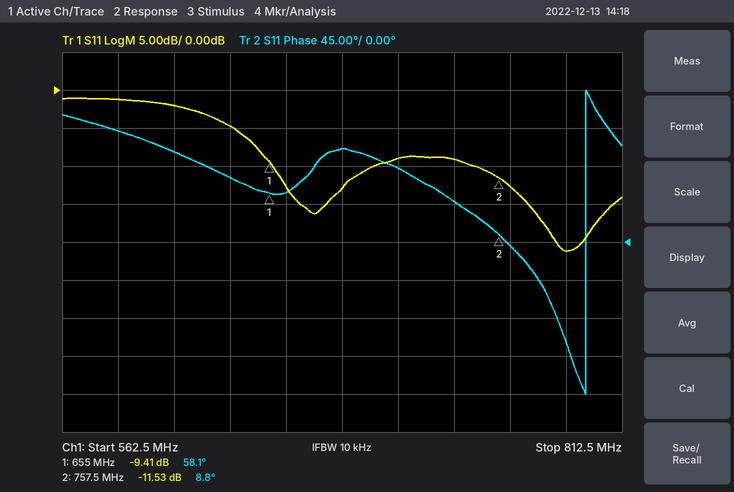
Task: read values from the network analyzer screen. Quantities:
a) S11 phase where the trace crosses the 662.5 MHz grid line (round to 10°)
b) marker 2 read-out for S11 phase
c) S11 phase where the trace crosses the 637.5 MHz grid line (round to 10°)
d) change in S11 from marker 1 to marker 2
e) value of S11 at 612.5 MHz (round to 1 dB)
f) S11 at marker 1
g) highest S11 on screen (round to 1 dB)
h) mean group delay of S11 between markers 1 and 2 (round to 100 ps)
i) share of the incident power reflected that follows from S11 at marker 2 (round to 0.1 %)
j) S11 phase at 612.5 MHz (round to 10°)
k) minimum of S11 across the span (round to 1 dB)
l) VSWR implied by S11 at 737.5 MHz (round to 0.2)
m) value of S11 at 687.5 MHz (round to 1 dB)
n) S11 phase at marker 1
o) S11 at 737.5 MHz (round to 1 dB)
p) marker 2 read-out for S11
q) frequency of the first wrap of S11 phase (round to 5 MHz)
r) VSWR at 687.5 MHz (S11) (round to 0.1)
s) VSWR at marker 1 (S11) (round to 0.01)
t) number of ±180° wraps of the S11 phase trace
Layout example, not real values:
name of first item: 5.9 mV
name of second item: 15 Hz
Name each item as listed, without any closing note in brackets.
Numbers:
S11 phase where the trace crosses the 662.5 MHz grid line: 60°
marker 2 read-out for S11 phase: 8.8°
S11 phase where the trace crosses the 637.5 MHz grid line: 80°
change in S11 from marker 1 to marker 2: -2.12 dB
value of S11 at 612.5 MHz: -2 dB
S11 at marker 1: -9.41 dB
highest S11 on screen: -1 dB
mean group delay of S11 between markers 1 and 2: 1.3 ns
share of the incident power reflected that follows from S11 at marker 2: 7.0 %
S11 phase at 612.5 MHz: 110°
minimum of S11 across the span: -21 dB
VSWR implied by S11 at 737.5 MHz: 2.0
value of S11 at 687.5 MHz: -13 dB
S11 phase at marker 1: 58.1°
S11 at 737.5 MHz: -9 dB
marker 2 read-out for S11: -11.53 dB
frequency of the first wrap of S11 phase: 795 MHz
VSWR at 687.5 MHz (S11): 1.6
VSWR at marker 1 (S11): 2.02
number of ±180° wraps of the S11 phase trace: 1
